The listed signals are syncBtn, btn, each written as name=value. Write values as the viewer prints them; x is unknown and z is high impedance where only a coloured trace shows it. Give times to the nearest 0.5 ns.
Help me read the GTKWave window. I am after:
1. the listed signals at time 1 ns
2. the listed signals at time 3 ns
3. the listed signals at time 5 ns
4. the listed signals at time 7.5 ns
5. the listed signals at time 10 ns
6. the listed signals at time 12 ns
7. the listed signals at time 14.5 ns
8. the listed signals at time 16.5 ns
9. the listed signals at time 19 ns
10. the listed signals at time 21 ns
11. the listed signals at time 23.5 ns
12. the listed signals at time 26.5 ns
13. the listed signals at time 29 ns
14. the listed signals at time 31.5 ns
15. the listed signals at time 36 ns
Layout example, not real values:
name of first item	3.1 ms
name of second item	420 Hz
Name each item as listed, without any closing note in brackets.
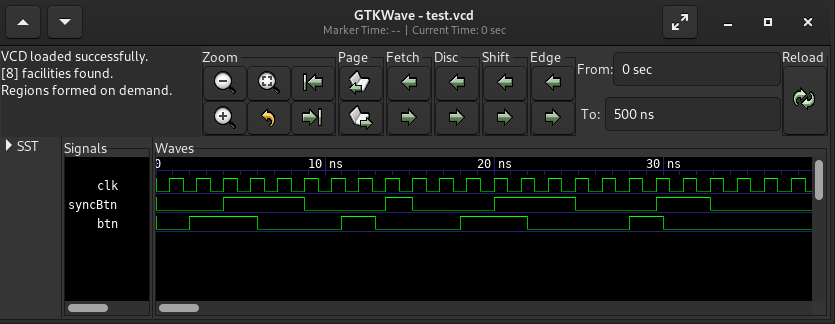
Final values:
the listed signals at time 1 ns	syncBtn=0, btn=0
the listed signals at time 3 ns	syncBtn=0, btn=1
the listed signals at time 5 ns	syncBtn=1, btn=1
the listed signals at time 7.5 ns	syncBtn=1, btn=0
the listed signals at time 10 ns	syncBtn=0, btn=0
the listed signals at time 12 ns	syncBtn=0, btn=1
the listed signals at time 14.5 ns	syncBtn=1, btn=0
the listed signals at time 16.5 ns	syncBtn=0, btn=0
the listed signals at time 19 ns	syncBtn=0, btn=1
the listed signals at time 21 ns	syncBtn=1, btn=1
the listed signals at time 23.5 ns	syncBtn=1, btn=0
the listed signals at time 26.5 ns	syncBtn=0, btn=0
the listed signals at time 29 ns	syncBtn=0, btn=1
the listed signals at time 31.5 ns	syncBtn=1, btn=0
the listed signals at time 36 ns	syncBtn=0, btn=0
